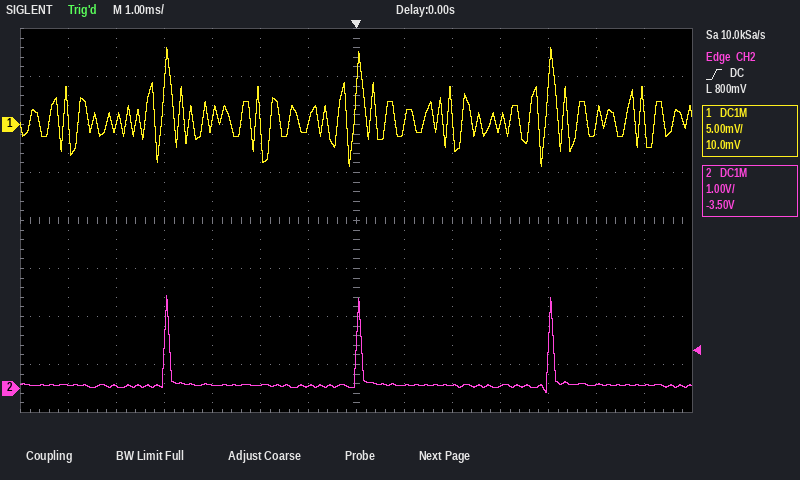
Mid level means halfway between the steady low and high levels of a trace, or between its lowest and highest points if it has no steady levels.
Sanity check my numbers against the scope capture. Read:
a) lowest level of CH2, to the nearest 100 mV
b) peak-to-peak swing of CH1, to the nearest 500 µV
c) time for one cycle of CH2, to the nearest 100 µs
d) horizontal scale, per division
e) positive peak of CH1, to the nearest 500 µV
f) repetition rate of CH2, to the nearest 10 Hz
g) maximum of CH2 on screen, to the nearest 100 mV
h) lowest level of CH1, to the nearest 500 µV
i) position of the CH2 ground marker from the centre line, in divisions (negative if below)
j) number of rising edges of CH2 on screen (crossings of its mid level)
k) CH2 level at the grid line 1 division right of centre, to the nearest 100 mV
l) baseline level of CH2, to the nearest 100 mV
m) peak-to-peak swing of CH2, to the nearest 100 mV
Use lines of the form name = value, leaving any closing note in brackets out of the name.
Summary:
lowest level of CH2, to the nearest 100 mV = -100 mV
peak-to-peak swing of CH1, to the nearest 500 µV = 12.5 mV
time for one cycle of CH2, to the nearest 100 µs = 4.0 ms
horizontal scale, per division = 1 ms
positive peak of CH1, to the nearest 500 µV = 8.0 mV
repetition rate of CH2, to the nearest 10 Hz = 250 Hz
maximum of CH2 on screen, to the nearest 100 mV = 1.9 V
lowest level of CH1, to the nearest 500 µV = -4.5 mV
position of the CH2 ground marker from the centre line, in divisions = -3.5 div
number of rising edges of CH2 on screen = 3
CH2 level at the grid line 1 division right of centre, to the nearest 100 mV = 100 mV
baseline level of CH2, to the nearest 100 mV = 100 mV
peak-to-peak swing of CH2, to the nearest 100 mV = 2.0 V
